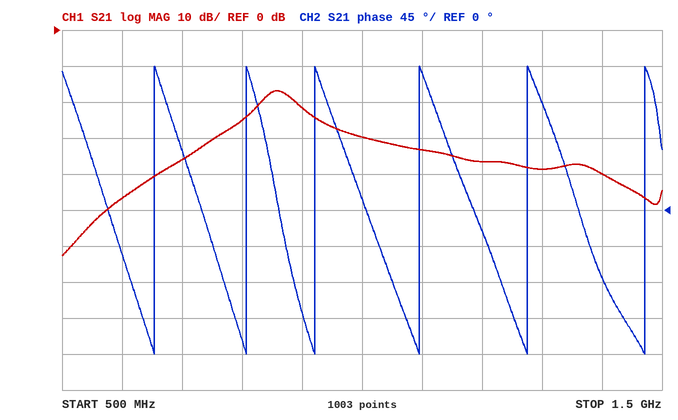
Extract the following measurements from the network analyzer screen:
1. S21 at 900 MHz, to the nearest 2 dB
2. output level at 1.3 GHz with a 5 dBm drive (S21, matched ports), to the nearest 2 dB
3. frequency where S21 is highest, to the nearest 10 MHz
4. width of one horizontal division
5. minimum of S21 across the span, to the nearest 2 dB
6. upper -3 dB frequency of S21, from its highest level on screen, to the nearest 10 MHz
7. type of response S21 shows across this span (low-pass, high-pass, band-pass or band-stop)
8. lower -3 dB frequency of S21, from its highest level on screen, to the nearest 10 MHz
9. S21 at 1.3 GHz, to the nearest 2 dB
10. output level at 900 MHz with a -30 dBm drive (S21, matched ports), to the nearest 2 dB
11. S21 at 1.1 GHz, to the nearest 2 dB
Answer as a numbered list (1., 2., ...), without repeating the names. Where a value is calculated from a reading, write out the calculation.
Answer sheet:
1. -22 dB
2. 5 dBm + (-38 dB) = -34 dBm
3. 860 MHz
4. 100 MHz
5. -62 dB
6. 890 MHz
7. band-pass
8. 830 MHz
9. -38 dB
10. -30 dBm + (-22 dB) = -52 dBm
11. -34 dB
